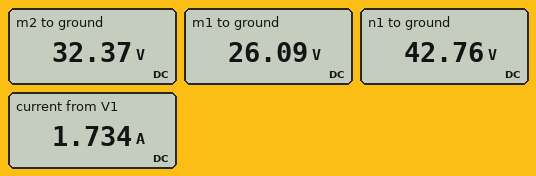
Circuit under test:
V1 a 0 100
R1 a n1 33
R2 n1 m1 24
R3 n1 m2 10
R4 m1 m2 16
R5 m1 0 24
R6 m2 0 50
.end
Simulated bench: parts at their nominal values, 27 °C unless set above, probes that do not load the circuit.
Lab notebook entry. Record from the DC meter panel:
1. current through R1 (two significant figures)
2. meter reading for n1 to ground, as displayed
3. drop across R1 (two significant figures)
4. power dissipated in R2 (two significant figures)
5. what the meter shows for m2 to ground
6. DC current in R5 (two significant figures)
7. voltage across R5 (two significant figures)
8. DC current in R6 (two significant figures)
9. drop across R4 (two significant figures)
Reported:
1.7 A
42.76 V
57 V
12 W
32.37 V
1.1 A
26 V
650 mA
6.3 V
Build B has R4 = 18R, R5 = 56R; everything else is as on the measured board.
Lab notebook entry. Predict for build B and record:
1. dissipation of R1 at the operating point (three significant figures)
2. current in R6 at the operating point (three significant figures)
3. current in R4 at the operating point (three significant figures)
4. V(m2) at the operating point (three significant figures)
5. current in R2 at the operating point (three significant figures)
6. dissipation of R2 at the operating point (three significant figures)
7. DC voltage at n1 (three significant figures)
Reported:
73.9 W
817 mA
156 mA
40.9 V
523 mA
6.57 W
50.6 V
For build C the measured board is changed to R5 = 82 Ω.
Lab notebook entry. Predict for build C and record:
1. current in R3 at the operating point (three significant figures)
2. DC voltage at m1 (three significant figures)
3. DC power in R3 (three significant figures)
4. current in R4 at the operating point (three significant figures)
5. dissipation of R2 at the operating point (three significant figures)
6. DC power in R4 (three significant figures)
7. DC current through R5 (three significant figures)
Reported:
956 mA
42.9 V
9.15 W
74.7 mA
4.82 W
89.3 mW
523 mA
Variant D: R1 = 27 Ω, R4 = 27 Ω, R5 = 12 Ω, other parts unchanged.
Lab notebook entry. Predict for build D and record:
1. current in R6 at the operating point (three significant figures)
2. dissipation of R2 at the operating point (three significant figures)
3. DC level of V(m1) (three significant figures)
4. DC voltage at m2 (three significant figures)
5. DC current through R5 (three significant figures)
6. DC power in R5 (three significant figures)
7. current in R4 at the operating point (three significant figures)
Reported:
626 mA
24.8 W
18.1 V
31.3 V
1.51 A
27.2 W
490 mA
